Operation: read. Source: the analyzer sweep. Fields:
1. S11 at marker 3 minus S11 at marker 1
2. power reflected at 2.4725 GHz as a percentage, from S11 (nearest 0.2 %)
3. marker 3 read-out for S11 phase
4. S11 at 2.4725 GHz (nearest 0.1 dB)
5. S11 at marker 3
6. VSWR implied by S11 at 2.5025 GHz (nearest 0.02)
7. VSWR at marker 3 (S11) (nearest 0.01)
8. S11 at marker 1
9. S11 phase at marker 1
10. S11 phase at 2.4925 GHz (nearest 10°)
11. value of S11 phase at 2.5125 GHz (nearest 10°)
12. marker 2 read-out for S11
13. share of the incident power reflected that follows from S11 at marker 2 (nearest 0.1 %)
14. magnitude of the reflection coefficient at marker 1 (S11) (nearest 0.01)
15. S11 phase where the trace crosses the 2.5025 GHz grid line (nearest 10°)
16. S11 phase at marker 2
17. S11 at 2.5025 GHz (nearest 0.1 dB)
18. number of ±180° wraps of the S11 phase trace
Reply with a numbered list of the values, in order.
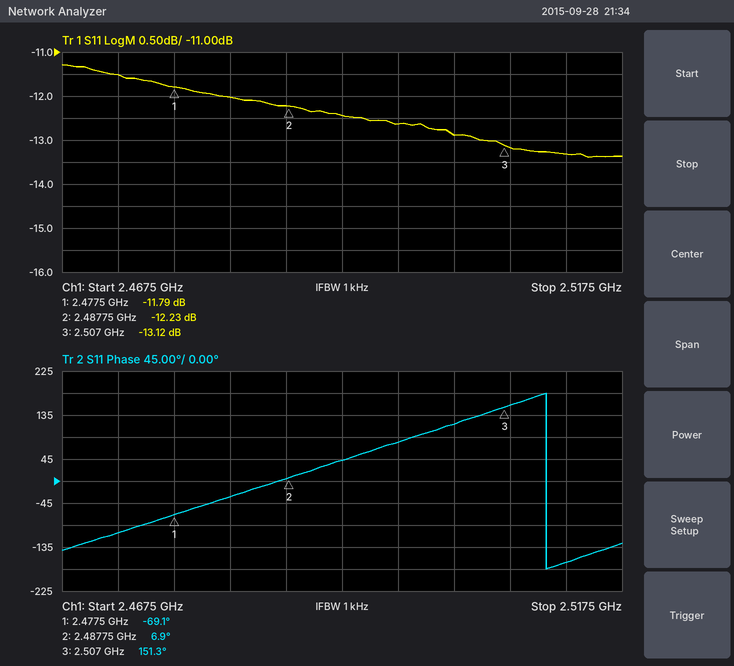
1. -1.33 dB
2. 7.0 %
3. 151.3°
4. -11.5 dB
5. -13.12 dB
6. 1.58
7. 1.57
8. -11.79 dB
9. -69.1°
10. 40°
11. -170°
12. -12.23 dB
13. 6.0 %
14. 0.26
15. 120°
16. 6.9°
17. -12.9 dB
18. 1
